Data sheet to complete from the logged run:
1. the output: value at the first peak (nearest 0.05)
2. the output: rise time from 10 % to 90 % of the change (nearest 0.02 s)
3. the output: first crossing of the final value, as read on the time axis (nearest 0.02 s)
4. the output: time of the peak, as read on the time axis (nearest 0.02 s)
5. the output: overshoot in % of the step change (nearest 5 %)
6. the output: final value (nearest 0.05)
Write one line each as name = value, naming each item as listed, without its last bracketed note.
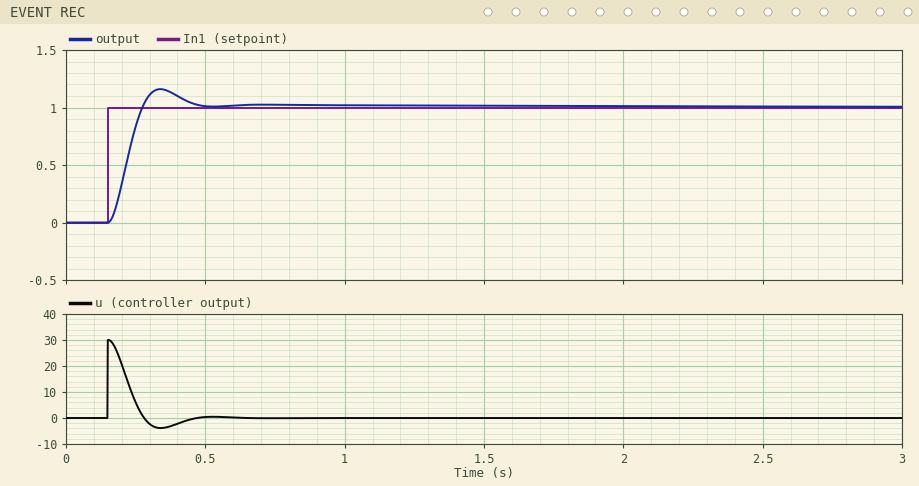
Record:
the output: value at the first peak = 1.15
the output: rise time from 10 % to 90 % of the change = 0.08 s
the output: first crossing of the final value, as read on the time axis = 0.28 s
the output: time of the peak, as read on the time axis = 0.34 s
the output: overshoot in % of the step change = 15 %
the output: final value = 1.00
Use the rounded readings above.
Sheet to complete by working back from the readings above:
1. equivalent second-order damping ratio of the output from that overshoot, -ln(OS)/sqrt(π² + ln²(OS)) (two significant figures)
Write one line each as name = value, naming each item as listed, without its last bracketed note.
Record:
equivalent second-order damping ratio of the output from that overshoot, -ln(OS)/sqrt(π² + ln²(OS)) = 0.52
